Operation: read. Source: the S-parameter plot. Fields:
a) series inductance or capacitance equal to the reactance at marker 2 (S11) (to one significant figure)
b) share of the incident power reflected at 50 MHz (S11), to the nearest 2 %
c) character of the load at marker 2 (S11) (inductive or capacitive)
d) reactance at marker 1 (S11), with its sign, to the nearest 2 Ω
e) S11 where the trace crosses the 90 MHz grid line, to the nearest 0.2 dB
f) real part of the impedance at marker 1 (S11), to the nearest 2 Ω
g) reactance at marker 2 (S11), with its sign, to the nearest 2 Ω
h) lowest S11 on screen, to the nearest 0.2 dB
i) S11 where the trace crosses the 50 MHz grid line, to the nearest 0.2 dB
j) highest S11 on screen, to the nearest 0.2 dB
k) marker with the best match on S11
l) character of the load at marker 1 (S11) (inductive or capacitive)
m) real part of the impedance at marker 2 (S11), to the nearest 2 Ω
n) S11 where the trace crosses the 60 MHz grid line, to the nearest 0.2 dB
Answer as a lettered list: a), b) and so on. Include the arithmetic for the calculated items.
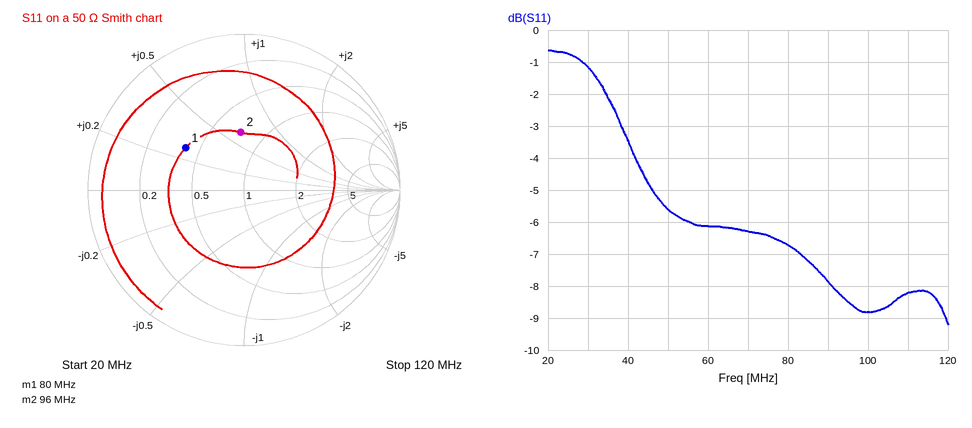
a) L = 32 Ω/(2π × 96 MHz) ≈ 53.1 nH, so 50 nH to one significant figure
b) 10^(-5.6/10) ≈ 28 %
c) inductive
d) +14 Ω
e) -7.8 dB
f) 20 Ω
g) +32 Ω
h) -9.2 dB
i) -5.6 dB
j) -0.6 dB
k) marker 2
l) inductive
m) 36 Ω
n) -6.2 dB
